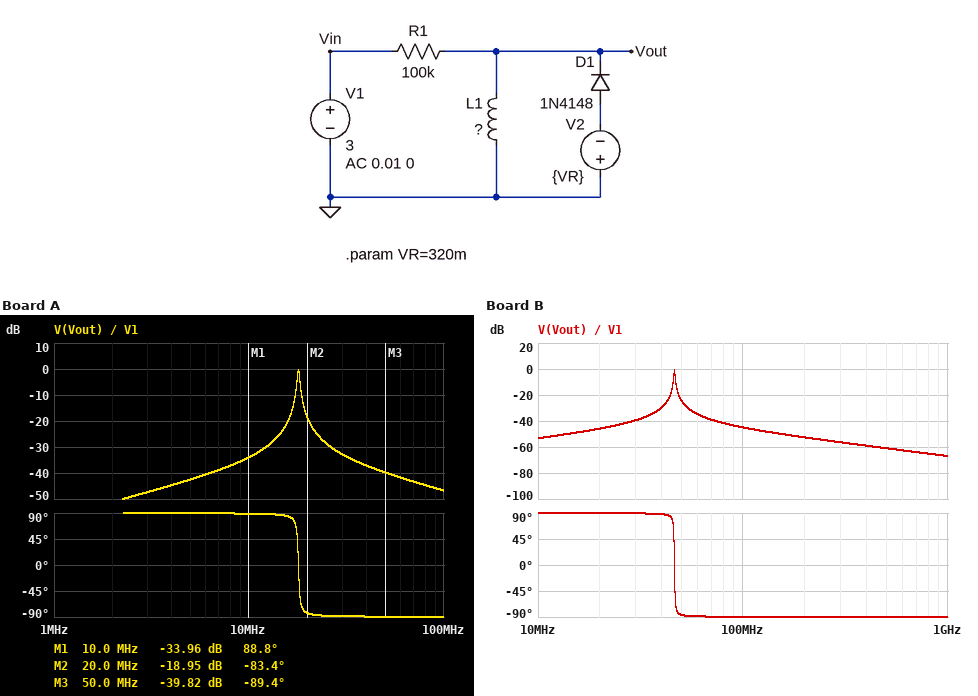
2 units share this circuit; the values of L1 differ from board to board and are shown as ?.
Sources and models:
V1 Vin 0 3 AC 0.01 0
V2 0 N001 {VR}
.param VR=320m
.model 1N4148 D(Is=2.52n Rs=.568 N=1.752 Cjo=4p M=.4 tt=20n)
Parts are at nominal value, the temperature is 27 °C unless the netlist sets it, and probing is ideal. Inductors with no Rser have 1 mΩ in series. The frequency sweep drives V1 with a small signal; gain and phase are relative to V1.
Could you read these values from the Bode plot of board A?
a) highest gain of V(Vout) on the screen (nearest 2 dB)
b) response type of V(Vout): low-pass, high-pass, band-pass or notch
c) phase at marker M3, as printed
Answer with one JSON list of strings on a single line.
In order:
["0 dB", "band-pass", "-89.4 deg"]
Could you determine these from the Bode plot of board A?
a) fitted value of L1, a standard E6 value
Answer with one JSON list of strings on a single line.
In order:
["22 µH"]
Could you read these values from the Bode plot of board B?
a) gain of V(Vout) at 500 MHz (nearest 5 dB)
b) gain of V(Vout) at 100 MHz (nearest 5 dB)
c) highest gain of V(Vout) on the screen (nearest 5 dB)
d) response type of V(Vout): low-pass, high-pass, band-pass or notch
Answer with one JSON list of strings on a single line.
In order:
["-60 dB", "-45 dB", "0 dB", "band-pass"]
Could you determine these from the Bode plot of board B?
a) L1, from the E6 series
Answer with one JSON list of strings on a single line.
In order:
["3.3 µH"]
